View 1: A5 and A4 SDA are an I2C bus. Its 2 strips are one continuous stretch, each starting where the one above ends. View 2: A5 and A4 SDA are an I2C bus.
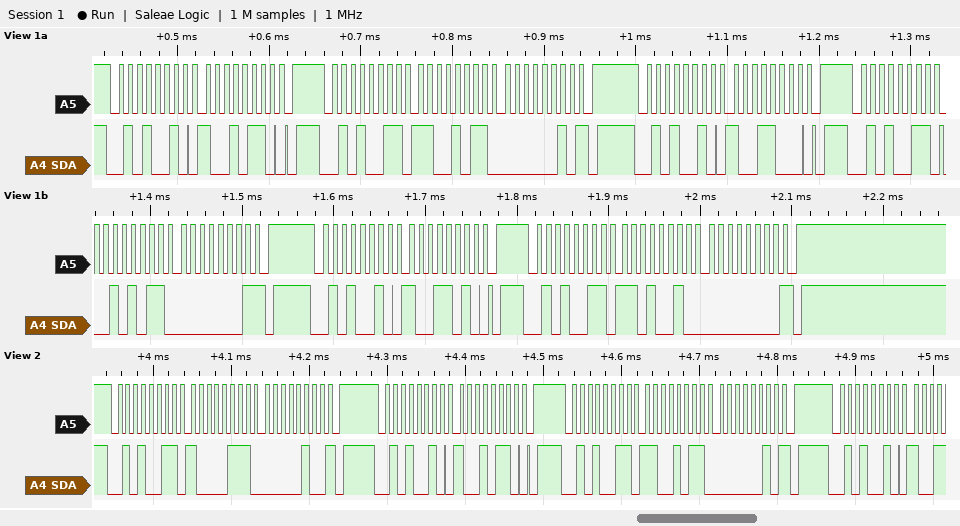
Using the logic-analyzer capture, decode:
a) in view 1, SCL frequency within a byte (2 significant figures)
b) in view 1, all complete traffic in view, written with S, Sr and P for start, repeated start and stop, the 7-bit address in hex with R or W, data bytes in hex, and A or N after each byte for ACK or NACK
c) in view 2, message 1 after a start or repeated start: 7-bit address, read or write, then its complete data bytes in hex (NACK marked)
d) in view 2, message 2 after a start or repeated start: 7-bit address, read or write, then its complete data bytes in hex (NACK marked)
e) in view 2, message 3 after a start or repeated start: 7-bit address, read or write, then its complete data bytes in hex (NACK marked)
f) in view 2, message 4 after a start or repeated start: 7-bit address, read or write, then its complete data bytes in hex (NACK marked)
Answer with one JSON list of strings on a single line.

["100 kHz", "S 29W A 96 A P S 29R A CB A 02 N P S 29W A 98 A P S 29R A 2B A 01 N P S 29W A 9A A P S 29R A D2 A 00 N P", "0x29 read: 87 04 NACK", "0x29 write: 96", "0x29 read: CB 02 NACK", "0x29 write"]
